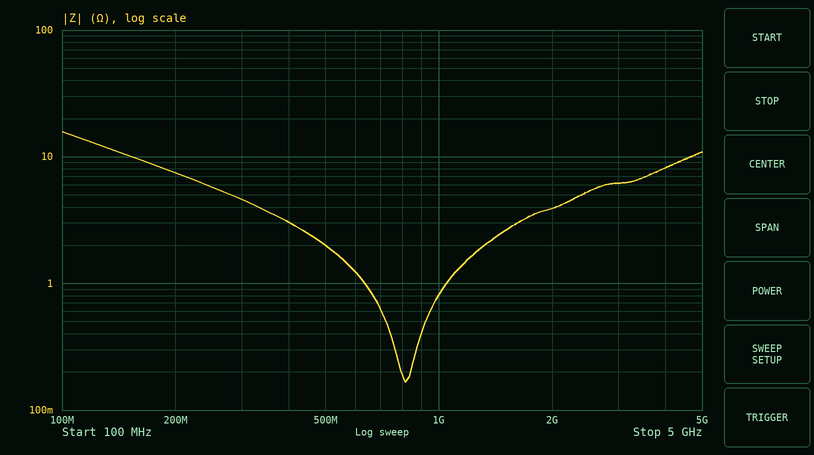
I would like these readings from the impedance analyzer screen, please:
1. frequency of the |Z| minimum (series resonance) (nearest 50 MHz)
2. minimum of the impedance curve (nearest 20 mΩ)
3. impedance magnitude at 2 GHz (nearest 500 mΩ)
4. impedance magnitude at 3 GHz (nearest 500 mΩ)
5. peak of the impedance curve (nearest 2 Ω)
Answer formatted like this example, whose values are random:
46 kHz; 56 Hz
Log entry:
800 MHz; 160 mΩ; 4.0 Ω; 6.0 Ω; 16 Ω
